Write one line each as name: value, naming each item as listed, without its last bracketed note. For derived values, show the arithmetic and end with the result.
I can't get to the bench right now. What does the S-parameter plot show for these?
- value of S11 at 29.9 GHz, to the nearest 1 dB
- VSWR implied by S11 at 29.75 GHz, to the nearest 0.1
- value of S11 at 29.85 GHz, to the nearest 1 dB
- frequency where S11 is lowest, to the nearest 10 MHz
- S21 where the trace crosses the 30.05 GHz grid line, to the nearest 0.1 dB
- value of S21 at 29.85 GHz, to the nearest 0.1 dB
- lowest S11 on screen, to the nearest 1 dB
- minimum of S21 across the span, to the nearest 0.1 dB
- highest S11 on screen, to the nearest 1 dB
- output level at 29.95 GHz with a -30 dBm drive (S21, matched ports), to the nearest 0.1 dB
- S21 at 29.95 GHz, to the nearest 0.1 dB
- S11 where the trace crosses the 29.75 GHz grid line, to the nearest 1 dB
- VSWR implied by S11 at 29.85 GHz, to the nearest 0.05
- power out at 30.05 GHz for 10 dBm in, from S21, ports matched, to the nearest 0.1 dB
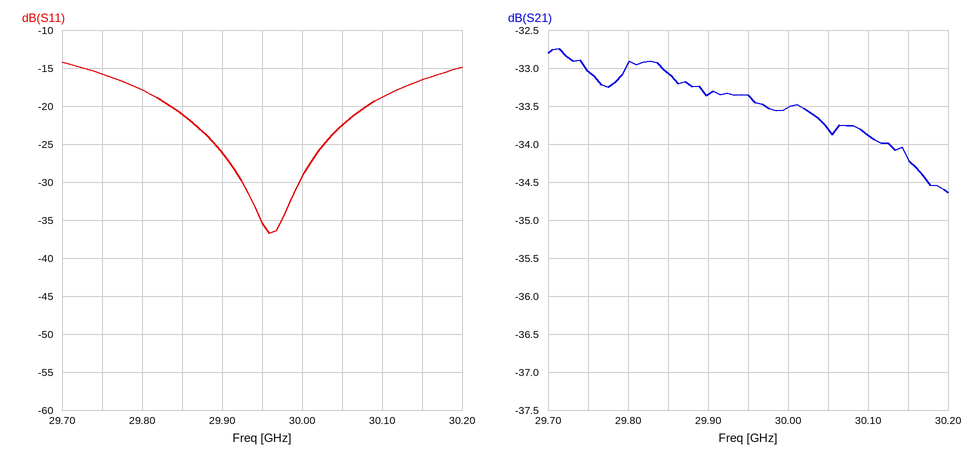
value of S11 at 29.9 GHz, to the nearest 1 dB: -26 dB
VSWR implied by S11 at 29.75 GHz, to the nearest 0.1: |Γ| = 10^(-16/20) = 0.1585; VSWR = (1 + 0.1585)/(1 − 0.1585) ≈ 1.4
value of S11 at 29.85 GHz, to the nearest 1 dB: -21 dB
frequency where S11 is lowest, to the nearest 10 MHz: 29.96 GHz
S21 where the trace crosses the 30.05 GHz grid line, to the nearest 0.1 dB: -33.8 dB
value of S21 at 29.85 GHz, to the nearest 0.1 dB: -33.1 dB
lowest S11 on screen, to the nearest 1 dB: -37 dB
minimum of S21 across the span, to the nearest 0.1 dB: -34.6 dB
highest S11 on screen, to the nearest 1 dB: -14 dB
output level at 29.95 GHz with a -30 dBm drive (S21, matched ports), to the nearest 0.1 dB: -30 dBm + (-33.4 dB) = -63.4 dBm
S21 at 29.95 GHz, to the nearest 0.1 dB: -33.4 dB
S11 where the trace crosses the 29.75 GHz grid line, to the nearest 1 dB: -16 dB
VSWR implied by S11 at 29.85 GHz, to the nearest 0.05: |Γ| = 10^(-21/20) = 0.0891; VSWR = (1 + 0.0891)/(1 − 0.0891) ≈ 1.20
power out at 30.05 GHz for 10 dBm in, from S21, ports matched, to the nearest 0.1 dB: 10 dBm + (-33.8 dB) = -23.8 dBm
